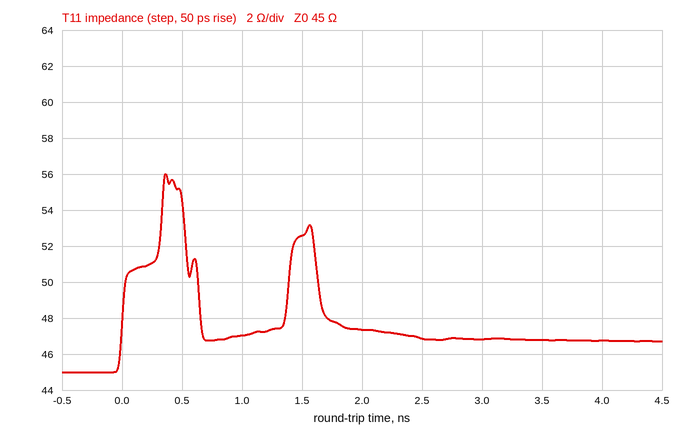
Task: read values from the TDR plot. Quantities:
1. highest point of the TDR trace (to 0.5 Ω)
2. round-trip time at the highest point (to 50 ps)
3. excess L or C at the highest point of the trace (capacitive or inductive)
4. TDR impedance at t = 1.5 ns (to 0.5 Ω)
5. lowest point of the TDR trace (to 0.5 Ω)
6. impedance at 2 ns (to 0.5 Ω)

56.0 Ω
350 ps
inductive
52.5 Ω
45.0 Ω
47.5 Ω
